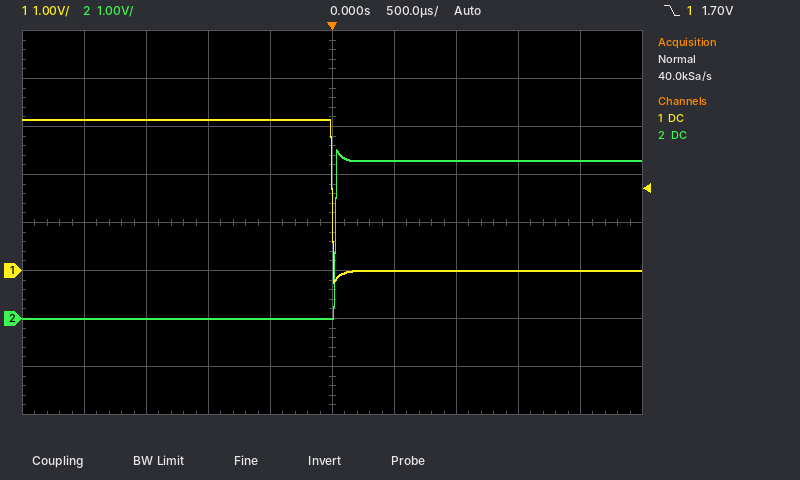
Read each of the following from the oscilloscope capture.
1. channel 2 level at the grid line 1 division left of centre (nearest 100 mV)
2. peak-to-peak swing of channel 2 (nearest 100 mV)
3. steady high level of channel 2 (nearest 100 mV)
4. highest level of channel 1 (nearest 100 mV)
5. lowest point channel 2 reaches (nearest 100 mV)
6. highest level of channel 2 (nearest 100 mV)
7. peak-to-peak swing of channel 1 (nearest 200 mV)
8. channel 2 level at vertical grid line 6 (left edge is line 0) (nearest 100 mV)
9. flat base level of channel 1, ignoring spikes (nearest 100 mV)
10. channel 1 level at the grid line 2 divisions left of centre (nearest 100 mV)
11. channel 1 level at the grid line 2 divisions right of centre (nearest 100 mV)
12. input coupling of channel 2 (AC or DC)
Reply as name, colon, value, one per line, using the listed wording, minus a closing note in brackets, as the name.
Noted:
channel 2 level at the grid line 1 division left of centre: 0.0 V
peak-to-peak swing of channel 2: 3.5 V
steady high level of channel 2: 3.3 V
highest level of channel 1: 3.1 V
lowest point channel 2 reaches: 0.0 V
highest level of channel 2: 3.5 V
peak-to-peak swing of channel 1: 3.4 V
channel 2 level at vertical grid line 6 (left edge is line 0): 3.3 V
flat base level of channel 1, ignoring spikes: 0.0 V
channel 1 level at the grid line 2 divisions left of centre: 3.1 V
channel 1 level at the grid line 2 divisions right of centre: 0.0 V
input coupling of channel 2: DC
